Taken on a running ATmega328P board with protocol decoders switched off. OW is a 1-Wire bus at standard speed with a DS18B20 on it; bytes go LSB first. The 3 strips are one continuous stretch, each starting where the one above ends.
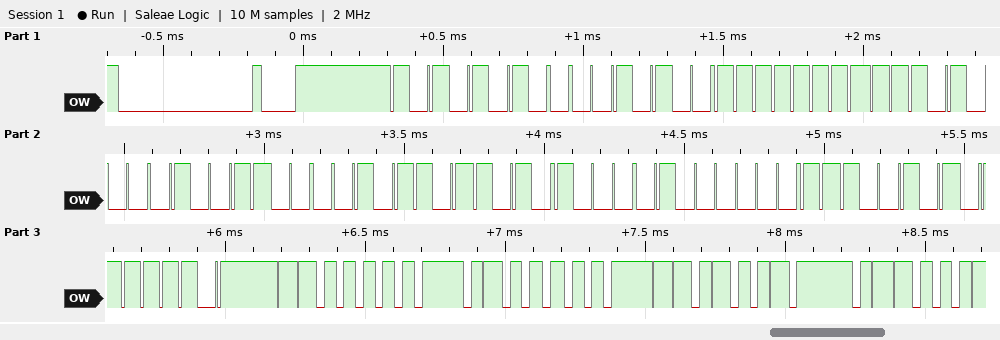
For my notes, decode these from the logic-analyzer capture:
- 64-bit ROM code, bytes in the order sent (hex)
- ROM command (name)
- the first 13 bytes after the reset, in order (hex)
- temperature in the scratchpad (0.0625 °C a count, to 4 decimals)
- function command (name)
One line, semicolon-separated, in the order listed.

28 FF 17 32 B4 15 02 A7; Match ROM; 55 28 FF 17 32 B4 15 02 A7 BE 03 02 4B; 32.1875 °C; Read Scratchpad
